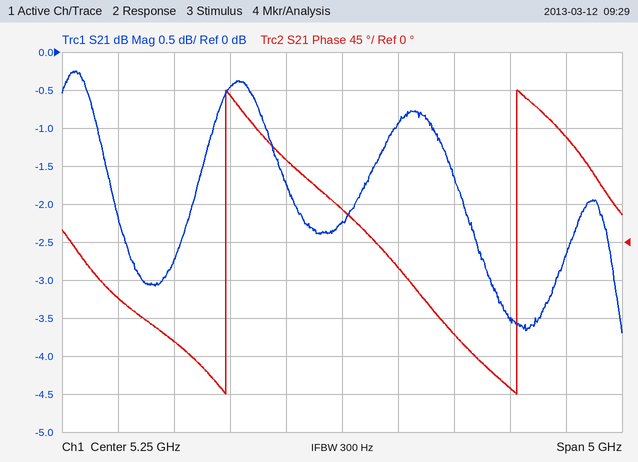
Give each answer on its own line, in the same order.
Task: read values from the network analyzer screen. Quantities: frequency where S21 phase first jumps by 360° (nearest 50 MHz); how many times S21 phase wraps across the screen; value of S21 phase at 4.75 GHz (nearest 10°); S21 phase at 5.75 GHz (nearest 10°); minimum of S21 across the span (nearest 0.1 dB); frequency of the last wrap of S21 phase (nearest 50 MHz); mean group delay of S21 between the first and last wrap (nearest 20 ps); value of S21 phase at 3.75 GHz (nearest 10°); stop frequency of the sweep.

4.20 GHz
2
100°
-30°
-3.7 dB
6.80 GHz
380 ps
-120°
7.75 GHz
